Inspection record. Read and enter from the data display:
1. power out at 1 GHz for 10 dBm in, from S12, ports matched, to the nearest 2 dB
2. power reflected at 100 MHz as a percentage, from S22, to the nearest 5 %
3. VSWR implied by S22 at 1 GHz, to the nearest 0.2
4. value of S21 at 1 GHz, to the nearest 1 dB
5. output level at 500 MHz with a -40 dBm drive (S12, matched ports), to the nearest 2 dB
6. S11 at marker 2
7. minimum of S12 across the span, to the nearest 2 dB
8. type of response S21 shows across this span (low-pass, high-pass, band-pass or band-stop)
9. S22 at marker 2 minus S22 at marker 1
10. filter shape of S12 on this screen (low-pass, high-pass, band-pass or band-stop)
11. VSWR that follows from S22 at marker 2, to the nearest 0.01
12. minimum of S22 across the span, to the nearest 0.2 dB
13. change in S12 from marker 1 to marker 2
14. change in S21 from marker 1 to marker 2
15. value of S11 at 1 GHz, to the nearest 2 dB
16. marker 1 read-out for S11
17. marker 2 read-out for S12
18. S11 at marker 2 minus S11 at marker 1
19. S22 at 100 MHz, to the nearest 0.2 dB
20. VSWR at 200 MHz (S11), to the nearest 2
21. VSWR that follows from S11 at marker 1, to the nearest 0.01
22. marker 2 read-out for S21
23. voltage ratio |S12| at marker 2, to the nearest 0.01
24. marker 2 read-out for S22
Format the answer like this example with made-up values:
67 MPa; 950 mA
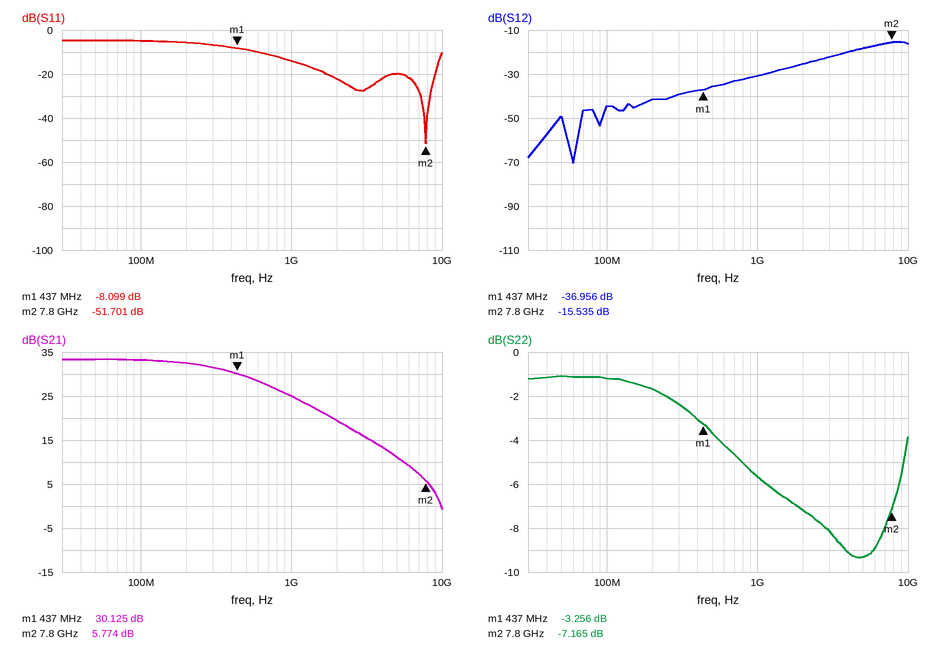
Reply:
-20 dBm; 75 %; 3.2; 25 dB; -76 dBm; -51.701 dB; -70 dB; low-pass; -3.909 dB; high-pass; 2.56; -9.4 dB; 21.421 dB; -24.351 dB; -14 dB; -8.099 dB; -15.535 dB; -43.602 dB; -1.2 dB; 4; 2.30; 5.774 dB; 0.17; -7.165 dB
